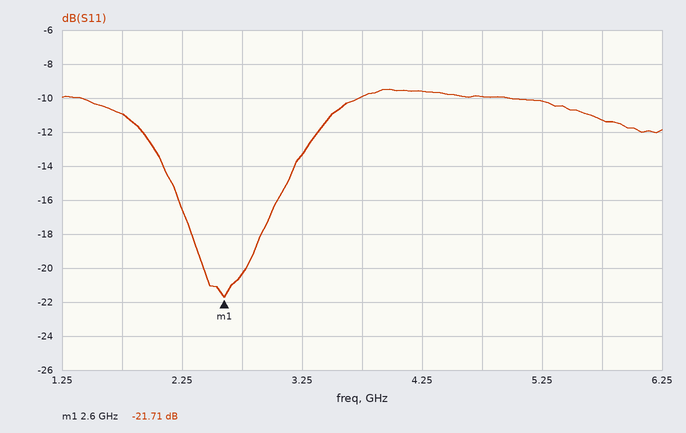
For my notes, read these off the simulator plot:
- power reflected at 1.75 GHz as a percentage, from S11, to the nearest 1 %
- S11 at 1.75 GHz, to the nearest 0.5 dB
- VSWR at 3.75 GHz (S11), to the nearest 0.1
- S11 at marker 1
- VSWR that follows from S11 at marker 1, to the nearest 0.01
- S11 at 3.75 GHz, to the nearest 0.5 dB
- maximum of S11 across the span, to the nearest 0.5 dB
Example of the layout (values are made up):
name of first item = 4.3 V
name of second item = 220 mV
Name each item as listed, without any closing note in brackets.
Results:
power reflected at 1.75 GHz as a percentage, from S11, to the nearest 1 % = 8 %
S11 at 1.75 GHz, to the nearest 0.5 dB = -11.0 dB
VSWR at 3.75 GHz (S11), to the nearest 0.1 = 1.9
S11 at marker 1 = -21.71 dB
VSWR that follows from S11 at marker 1, to the nearest 0.01 = 1.18
S11 at 3.75 GHz, to the nearest 0.5 dB = -10.0 dB
maximum of S11 across the span, to the nearest 0.5 dB = -9.5 dB
